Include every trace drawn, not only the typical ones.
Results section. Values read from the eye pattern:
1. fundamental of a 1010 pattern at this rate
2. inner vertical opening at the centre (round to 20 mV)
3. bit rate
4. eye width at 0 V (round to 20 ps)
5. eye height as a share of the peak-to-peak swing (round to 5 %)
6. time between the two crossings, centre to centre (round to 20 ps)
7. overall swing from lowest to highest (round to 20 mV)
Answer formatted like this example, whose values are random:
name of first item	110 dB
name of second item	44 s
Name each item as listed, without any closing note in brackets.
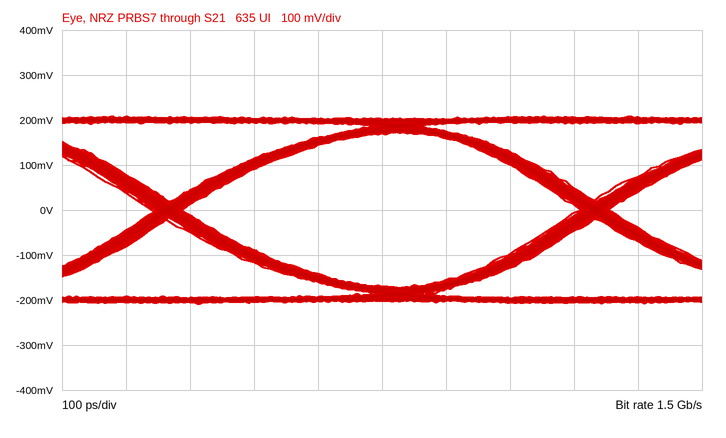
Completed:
fundamental of a 1010 pattern at this rate	750 MHz
inner vertical opening at the centre	340 mV
bit rate	1.5 Gb/s
eye width at 0 V	620 ps
eye height as a share of the peak-to-peak swing	80 %
time between the two crossings, centre to centre	660 ps
overall swing from lowest to highest	420 mV
